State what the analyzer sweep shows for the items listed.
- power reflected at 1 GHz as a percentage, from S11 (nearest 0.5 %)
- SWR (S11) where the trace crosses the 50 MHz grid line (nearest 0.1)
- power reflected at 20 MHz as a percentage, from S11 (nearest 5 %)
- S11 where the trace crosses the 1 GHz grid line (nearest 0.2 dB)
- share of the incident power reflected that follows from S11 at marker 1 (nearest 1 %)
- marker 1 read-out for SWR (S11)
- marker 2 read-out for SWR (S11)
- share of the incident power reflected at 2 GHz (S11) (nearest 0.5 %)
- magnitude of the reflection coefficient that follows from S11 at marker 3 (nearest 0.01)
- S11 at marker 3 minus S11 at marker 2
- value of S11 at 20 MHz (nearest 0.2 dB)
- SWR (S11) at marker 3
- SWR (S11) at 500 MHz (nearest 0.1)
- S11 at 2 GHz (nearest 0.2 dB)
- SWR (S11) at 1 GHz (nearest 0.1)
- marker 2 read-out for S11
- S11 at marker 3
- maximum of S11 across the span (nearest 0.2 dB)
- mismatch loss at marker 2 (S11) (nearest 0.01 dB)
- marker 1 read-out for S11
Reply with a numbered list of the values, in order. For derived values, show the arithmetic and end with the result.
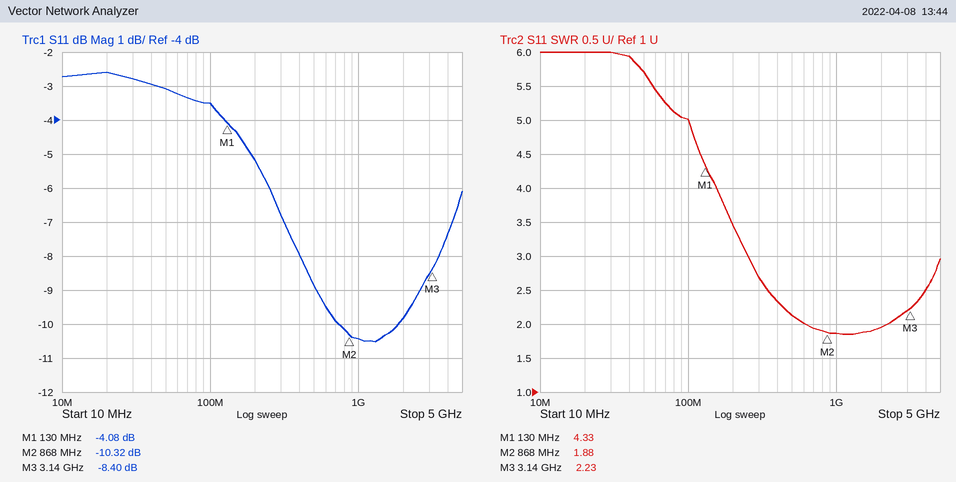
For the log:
1. 10^(-10.4/10) ≈ 9.12 %, so 9.0 % to the nearest 0.5 %
2. 5.7
3. 10^(-2.6/10) ≈ 55 %
4. -10.4 dB
5. 10^(-4.08/10) ≈ 39 %
6. 4.33
7. 1.88
8. 10^(-9.8/10) ≈ 10.5 %
9. 10^(-8.4/20) ≈ 0.38
10. -8.4 − (-10.32) = 1.92 dB
11. -2.6 dB
12. 2.23
13. 2.1
14. -9.8 dB
15. 1.9
16. -10.32 dB
17. -8.40 dB
18. -2.6 dB
19. −10 log10(1 − 10^(-10.32/10)) ≈ 0.42 dB
20. -4.08 dB
